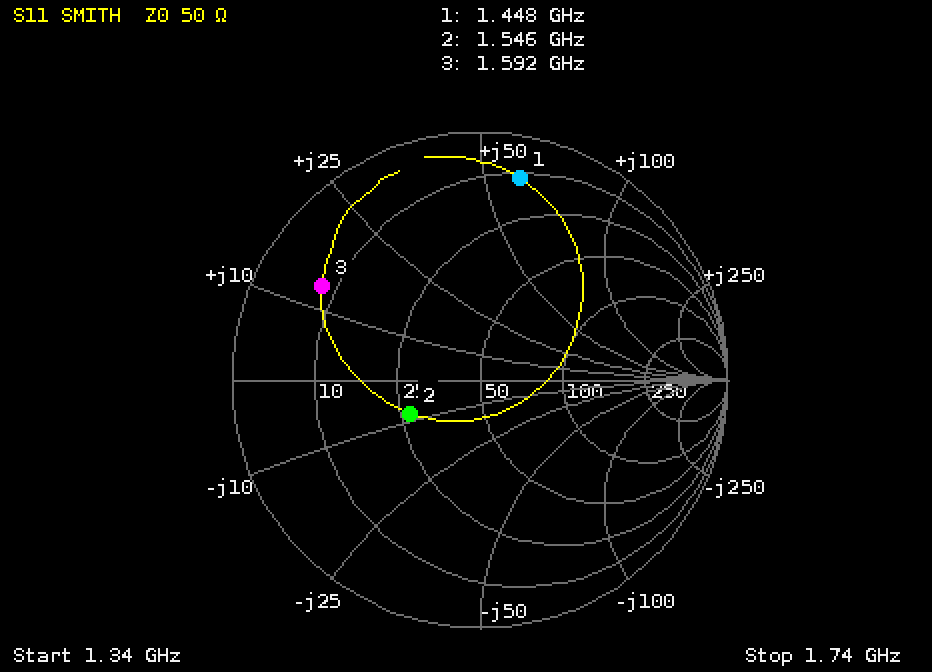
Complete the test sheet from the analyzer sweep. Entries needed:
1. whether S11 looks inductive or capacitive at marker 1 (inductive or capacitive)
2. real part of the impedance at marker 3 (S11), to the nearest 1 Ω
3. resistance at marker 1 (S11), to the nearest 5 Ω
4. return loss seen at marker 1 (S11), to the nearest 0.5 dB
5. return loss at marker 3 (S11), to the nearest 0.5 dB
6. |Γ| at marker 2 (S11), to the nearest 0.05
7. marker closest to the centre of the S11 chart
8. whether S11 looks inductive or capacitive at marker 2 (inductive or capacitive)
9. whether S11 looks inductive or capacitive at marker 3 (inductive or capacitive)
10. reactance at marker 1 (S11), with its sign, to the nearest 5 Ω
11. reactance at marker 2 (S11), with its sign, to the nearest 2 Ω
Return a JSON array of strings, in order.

["inductive", "8 Ω", "10 Ω", "1.5 dB", "2.5 dB", "0.30", "marker 2", "capacitive", "inductive", "+60 Ω", "-8 Ω"]
